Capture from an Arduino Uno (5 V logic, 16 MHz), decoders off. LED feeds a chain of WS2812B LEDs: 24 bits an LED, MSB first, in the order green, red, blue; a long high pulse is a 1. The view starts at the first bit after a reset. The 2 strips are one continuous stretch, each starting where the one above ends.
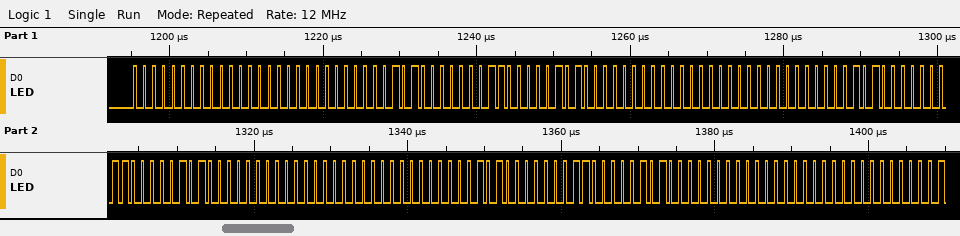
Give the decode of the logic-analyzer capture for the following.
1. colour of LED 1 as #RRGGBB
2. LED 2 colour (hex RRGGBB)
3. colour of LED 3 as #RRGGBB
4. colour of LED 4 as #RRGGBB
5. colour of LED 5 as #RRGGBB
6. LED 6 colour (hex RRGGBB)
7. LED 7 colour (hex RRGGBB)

#000000
#06140A
#000000
#06140A
#000000
#06140A
#000000
